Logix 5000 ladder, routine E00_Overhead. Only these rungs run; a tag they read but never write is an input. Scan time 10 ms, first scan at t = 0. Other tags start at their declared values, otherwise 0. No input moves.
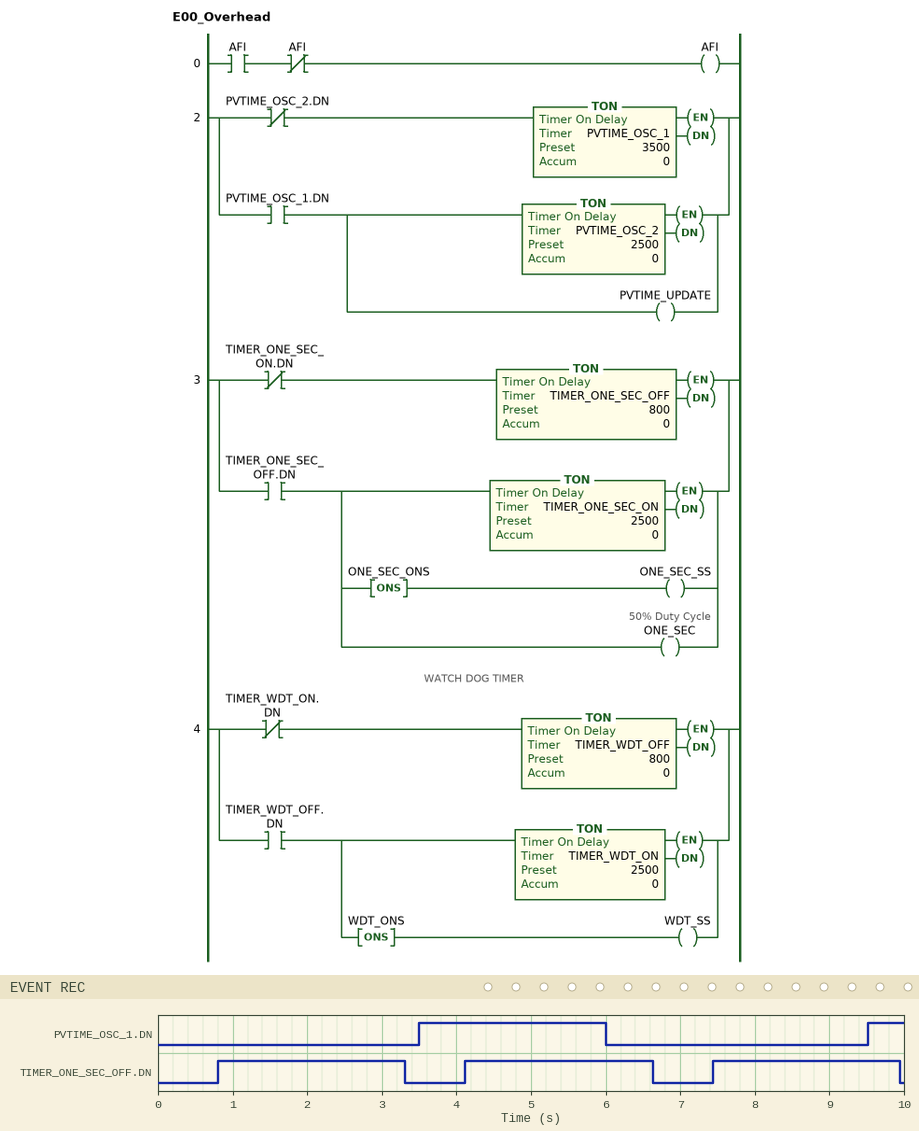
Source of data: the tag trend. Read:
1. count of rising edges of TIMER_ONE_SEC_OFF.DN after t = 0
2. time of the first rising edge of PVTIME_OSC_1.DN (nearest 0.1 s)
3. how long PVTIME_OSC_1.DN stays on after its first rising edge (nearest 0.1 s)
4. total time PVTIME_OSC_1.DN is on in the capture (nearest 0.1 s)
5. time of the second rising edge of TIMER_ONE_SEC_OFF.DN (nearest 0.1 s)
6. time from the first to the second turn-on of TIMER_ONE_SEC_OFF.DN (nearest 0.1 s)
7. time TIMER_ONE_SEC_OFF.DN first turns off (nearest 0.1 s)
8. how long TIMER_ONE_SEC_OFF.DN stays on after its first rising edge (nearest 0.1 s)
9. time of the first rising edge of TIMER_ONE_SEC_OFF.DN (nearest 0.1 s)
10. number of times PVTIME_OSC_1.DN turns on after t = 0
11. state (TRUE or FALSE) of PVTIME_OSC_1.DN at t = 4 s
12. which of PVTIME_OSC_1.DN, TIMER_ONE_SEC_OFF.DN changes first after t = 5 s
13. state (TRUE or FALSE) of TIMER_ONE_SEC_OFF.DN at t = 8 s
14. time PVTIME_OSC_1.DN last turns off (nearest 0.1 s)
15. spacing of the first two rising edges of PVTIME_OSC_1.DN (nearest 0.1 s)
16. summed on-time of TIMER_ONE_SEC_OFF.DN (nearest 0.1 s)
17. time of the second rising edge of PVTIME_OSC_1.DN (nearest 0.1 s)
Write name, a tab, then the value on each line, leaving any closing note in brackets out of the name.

count of rising edges of TIMER_ONE_SEC_OFF.DN after t = 0	3
time of the first rising edge of PVTIME_OSC_1.DN	3.5 s
how long PVTIME_OSC_1.DN stays on after its first rising edge	2.5 s
total time PVTIME_OSC_1.DN is on in the capture	3.0 s
time of the second rising edge of TIMER_ONE_SEC_OFF.DN	4.1 s
time from the first to the second turn-on of TIMER_ONE_SEC_OFF.DN	3.3 s
time TIMER_ONE_SEC_OFF.DN first turns off	3.3 s
how long TIMER_ONE_SEC_OFF.DN stays on after its first rising edge	2.5 s
time of the first rising edge of TIMER_ONE_SEC_OFF.DN	0.8 s
number of times PVTIME_OSC_1.DN turns on after t = 0	2
state (TRUE or FALSE) of PVTIME_OSC_1.DN at t = 4 s	TRUE
which of PVTIME_OSC_1.DN, TIMER_ONE_SEC_OFF.DN changes first after t = 5 s	PVTIME_OSC_1.DN
state (TRUE or FALSE) of TIMER_ONE_SEC_OFF.DN at t = 8 s	TRUE
time PVTIME_OSC_1.DN last turns off	6.0 s
spacing of the first two rising edges of PVTIME_OSC_1.DN	6.0 s
summed on-time of TIMER_ONE_SEC_OFF.DN	7.5 s
time of the second rising edge of PVTIME_OSC_1.DN	9.5 s
